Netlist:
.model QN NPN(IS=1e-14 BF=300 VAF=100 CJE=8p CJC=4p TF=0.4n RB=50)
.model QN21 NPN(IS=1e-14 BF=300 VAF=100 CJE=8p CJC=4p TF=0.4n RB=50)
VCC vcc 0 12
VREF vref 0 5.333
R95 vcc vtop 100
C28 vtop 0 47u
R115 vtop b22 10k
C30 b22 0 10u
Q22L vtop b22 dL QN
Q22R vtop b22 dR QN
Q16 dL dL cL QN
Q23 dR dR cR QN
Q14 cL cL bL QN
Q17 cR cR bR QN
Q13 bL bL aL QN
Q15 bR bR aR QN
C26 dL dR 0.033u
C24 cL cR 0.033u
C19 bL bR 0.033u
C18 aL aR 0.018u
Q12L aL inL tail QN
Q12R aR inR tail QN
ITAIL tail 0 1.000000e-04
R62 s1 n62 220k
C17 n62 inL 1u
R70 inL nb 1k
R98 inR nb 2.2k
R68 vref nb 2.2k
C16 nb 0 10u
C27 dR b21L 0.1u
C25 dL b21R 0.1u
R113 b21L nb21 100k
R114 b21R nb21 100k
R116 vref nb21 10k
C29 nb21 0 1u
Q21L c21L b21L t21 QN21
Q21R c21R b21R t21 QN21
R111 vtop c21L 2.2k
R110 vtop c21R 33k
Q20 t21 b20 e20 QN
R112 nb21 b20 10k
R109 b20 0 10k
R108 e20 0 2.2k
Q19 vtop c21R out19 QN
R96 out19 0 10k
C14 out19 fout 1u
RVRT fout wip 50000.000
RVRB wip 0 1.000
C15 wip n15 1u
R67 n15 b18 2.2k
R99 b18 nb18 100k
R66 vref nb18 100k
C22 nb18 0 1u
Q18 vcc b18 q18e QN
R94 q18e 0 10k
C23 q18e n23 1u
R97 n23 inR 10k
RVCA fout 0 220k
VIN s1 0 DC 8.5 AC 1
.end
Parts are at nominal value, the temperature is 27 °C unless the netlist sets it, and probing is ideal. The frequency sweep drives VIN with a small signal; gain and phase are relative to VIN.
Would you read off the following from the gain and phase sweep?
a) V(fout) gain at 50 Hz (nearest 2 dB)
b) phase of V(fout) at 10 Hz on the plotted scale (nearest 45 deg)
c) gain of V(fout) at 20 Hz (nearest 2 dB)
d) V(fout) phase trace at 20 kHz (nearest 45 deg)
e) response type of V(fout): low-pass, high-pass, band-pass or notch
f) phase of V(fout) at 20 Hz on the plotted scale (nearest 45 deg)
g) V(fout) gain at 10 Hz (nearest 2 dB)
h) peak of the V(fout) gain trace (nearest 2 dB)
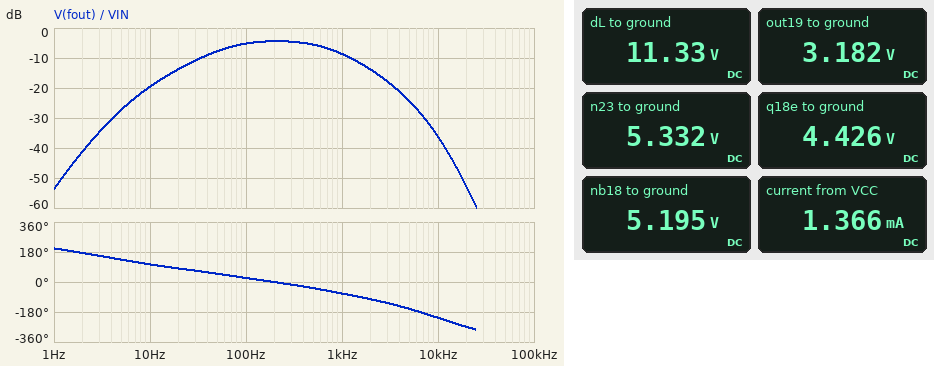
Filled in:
-8 dB
90 deg
-14 dB
-270 deg
band-pass
90 deg
-20 dB
-4 dB
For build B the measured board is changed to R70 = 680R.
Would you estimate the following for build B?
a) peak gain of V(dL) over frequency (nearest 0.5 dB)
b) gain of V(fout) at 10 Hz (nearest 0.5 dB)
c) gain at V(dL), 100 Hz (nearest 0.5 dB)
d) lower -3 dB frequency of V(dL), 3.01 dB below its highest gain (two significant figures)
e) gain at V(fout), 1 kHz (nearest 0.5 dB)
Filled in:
-54.0 dB
-22.5 dB
-56.5 dB
1.3 Hz
-12.0 dB
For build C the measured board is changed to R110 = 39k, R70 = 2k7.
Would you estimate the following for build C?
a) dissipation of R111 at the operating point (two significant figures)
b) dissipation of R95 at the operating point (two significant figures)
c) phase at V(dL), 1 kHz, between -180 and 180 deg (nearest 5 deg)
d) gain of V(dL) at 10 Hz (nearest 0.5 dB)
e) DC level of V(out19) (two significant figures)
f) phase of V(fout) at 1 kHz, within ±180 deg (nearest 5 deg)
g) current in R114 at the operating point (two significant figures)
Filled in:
170 µW
72 µW
90 deg
-44.0 dB
2.4 V
-30 deg
900 nA
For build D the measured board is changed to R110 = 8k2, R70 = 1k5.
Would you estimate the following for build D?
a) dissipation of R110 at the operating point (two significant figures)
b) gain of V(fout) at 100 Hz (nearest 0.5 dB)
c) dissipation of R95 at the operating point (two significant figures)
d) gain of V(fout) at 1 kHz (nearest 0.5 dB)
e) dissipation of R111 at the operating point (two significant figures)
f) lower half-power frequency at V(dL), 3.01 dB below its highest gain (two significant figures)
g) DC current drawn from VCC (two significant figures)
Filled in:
530 µW
-13.5 dB
230 µW
-17.0 dB
140 µW
890 mHz
2.0 mA
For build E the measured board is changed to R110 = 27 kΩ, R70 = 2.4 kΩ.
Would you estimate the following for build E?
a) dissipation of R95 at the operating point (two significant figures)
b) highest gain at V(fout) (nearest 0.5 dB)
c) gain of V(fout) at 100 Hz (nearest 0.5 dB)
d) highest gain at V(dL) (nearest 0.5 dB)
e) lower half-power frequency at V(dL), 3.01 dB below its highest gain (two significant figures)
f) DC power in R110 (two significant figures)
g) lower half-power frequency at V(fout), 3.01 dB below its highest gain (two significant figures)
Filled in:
110 µW
1.5 dB
0.5 dB
-44.5 dB
900 mHz
1.7 mW
54 Hz
